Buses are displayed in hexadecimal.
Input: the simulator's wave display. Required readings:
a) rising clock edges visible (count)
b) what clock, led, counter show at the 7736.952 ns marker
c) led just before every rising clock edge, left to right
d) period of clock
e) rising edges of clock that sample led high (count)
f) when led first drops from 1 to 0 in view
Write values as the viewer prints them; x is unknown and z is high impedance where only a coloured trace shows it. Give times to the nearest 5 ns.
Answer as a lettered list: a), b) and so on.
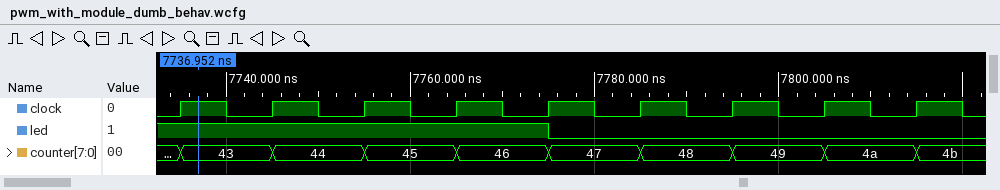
a) 9
b) clock=1, led=1, counter=43
c) 1 1 1 1 1 0 0 0 0
d) 10 ns
e) 5
f) 7775 ns
